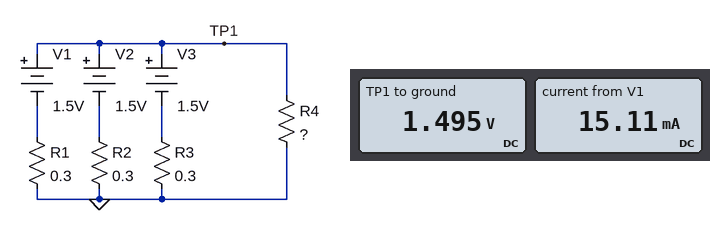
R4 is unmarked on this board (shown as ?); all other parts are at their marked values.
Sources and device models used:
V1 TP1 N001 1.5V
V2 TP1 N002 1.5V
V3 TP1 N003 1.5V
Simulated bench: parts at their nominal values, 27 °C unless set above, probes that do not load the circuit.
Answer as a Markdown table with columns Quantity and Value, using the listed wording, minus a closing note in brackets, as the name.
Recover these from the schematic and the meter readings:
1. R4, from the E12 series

| Quantity | Value |
|---|---|
| R4, from the E12 series | 33 Ω |
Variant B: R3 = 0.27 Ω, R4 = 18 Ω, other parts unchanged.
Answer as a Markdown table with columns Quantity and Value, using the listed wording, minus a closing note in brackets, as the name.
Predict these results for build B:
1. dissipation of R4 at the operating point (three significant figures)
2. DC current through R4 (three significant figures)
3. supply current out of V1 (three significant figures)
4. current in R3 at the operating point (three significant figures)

| Quantity | Value |
|---|---|
| dissipation of R4 at the operating point | 124 mW |
| DC current through R4 | 82.9 mA |
| supply current out of V1 | 26.6 mA |
| current in R3 at the operating point | 29.6 mA |
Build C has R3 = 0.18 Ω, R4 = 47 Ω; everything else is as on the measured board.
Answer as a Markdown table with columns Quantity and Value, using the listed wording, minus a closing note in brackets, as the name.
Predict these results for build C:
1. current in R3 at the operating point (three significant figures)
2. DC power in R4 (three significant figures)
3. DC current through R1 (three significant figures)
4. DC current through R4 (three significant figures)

| Quantity | Value |
|---|---|
| current in R3 at the operating point | 14.5 mA |
| DC power in R4 | 47.7 mW |
| DC current through R1 | 8.69 mA |
| DC current through R4 | 31.9 mA |
